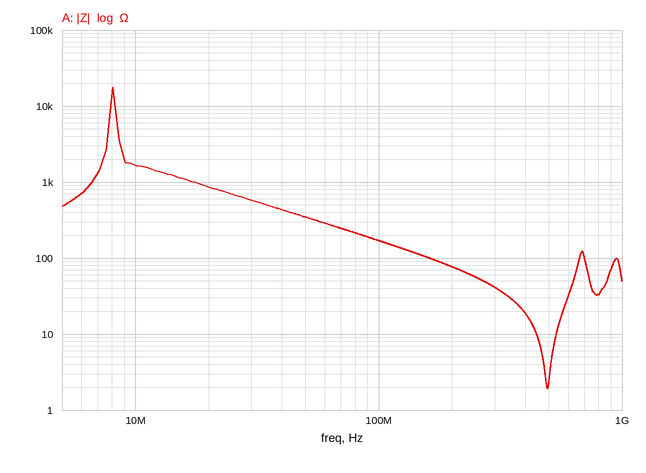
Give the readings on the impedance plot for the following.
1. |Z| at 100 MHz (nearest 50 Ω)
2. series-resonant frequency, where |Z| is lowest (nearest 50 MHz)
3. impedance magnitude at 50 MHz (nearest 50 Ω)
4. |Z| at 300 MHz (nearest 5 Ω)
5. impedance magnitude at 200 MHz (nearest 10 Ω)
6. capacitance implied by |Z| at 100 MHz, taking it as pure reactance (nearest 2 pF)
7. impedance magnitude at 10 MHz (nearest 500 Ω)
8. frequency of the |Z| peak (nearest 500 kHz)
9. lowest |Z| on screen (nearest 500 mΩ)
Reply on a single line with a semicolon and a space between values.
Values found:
150 Ω; 500 MHz; 350 Ω; 40 Ω; 80 Ω; 10 pF; 1.5 kΩ; 8.0 MHz; 2.0 Ω
